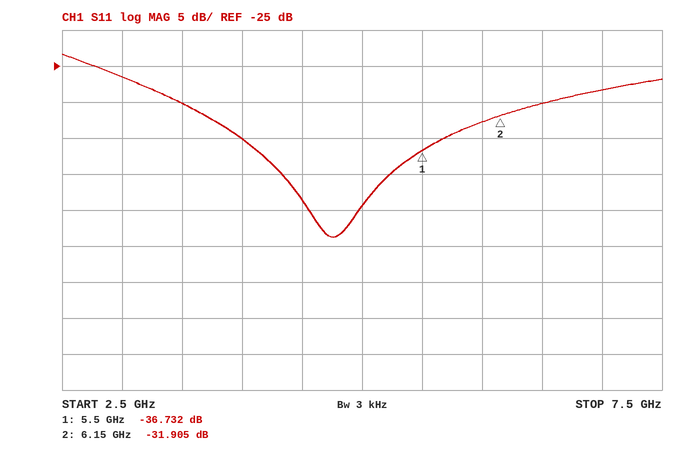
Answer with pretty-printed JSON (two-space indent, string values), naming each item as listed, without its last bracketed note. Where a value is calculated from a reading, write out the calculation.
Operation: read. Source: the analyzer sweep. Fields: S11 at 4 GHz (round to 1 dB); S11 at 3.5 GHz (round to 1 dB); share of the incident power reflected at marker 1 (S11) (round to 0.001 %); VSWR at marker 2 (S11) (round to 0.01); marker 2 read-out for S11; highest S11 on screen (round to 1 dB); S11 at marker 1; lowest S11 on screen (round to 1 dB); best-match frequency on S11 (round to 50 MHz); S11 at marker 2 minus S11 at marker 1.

{
  "S11 at 4 GHz": "-35 dB",
  "S11 at 3.5 GHz": "-30 dB",
  "share of the incident power reflected at marker 1 (S11)": "10^(-36.732/10) ≈ 0.021 %",
  "VSWR at marker 2 (S11)": "(1 + 0.0254)/(1 − 0.0254) ≈ 1.05",
  "marker 2 read-out for S11": "-31.905 dB",
  "highest S11 on screen": "-23 dB",
  "S11 at marker 1": "-36.732 dB",
  "lowest S11 on screen": "-49 dB",
  "best-match frequency on S11": "4.75 GHz",
  "S11 at marker 2 minus S11 at marker 1": "-31.905 − (-36.732) = 4.827 dB"
}
